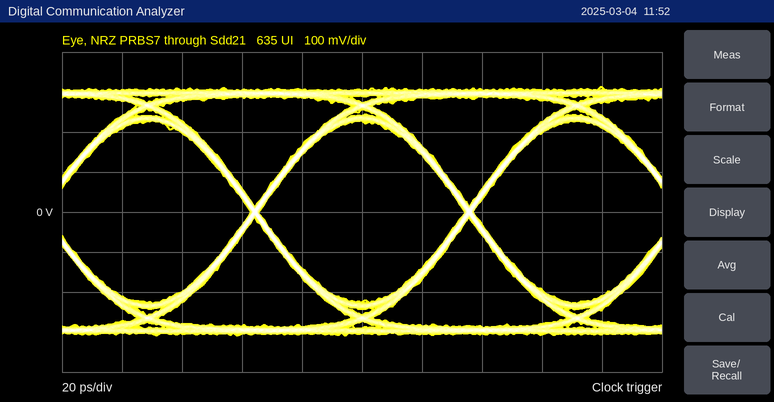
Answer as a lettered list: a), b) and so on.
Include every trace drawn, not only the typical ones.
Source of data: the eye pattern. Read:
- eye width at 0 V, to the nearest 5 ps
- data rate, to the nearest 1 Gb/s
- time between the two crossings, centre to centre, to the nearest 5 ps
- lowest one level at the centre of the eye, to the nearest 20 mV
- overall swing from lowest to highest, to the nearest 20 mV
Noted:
a) 70 ps
b) 14 Gb/s
c) 70 ps
d) 220 mV
e) 620 mV
